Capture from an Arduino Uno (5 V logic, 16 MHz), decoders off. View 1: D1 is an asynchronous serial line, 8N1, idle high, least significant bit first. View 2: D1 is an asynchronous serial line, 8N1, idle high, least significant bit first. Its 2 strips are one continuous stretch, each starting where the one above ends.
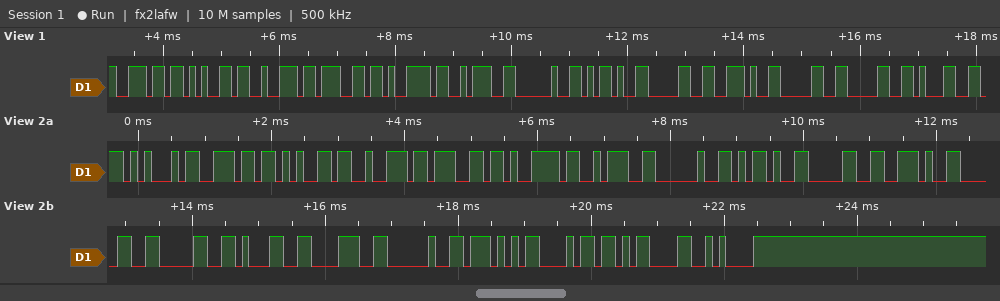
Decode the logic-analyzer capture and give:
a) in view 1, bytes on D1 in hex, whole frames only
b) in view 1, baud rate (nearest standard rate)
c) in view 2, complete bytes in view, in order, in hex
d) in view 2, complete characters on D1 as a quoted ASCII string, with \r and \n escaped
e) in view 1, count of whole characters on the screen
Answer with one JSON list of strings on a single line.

["6E 65 72 67 79 3A 20 2D 30 2E 30 30 31", "9600 baud", "45 6E 65 72 67 79 3A 20 2D 30 2E 30 30 31 38 20 57 68 0D 0A", "\"Energy: -0.0018 Wh\\r\\n\"", "13"]
